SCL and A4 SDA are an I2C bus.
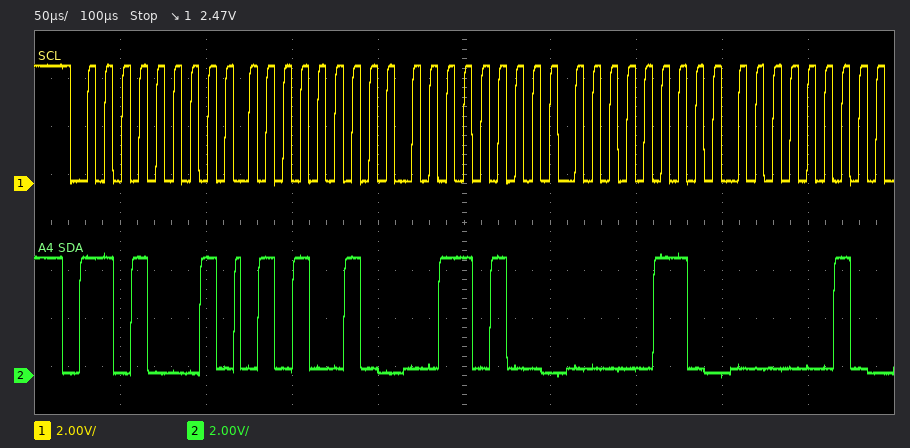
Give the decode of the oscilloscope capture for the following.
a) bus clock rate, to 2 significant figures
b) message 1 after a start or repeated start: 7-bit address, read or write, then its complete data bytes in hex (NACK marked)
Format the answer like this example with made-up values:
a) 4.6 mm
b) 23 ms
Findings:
a) 100 kHz
b) 0x68 read: 52 34 06 02
